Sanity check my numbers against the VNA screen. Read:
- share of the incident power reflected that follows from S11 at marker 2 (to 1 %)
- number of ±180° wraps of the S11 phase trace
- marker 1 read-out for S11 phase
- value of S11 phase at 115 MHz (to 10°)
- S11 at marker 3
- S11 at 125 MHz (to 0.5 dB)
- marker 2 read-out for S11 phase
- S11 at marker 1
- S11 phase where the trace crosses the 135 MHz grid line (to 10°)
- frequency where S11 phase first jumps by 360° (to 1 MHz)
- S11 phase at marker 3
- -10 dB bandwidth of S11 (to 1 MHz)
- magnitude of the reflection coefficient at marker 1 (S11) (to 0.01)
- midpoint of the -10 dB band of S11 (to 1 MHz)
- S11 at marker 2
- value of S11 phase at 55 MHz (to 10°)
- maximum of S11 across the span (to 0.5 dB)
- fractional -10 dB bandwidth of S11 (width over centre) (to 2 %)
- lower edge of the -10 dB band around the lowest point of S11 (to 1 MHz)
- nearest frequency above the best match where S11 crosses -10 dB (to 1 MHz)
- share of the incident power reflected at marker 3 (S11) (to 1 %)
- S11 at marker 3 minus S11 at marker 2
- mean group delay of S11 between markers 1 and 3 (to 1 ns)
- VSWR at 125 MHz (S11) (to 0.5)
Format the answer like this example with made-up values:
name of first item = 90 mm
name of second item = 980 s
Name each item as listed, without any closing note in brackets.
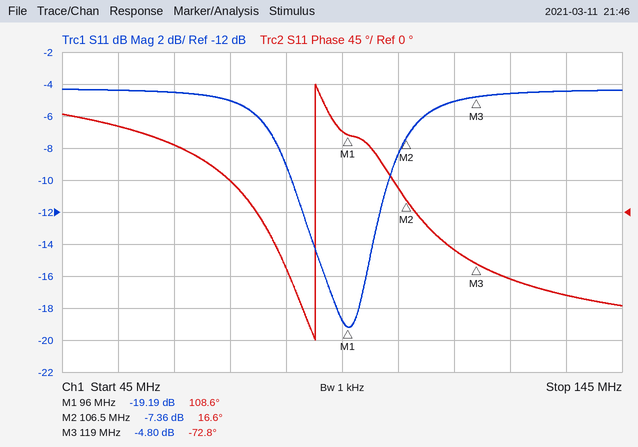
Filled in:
share of the incident power reflected that follows from S11 at marker 2 = 18 %
number of ±180° wraps of the S11 phase trace = 1
marker 1 read-out for S11 phase = 108.6°
value of S11 phase at 115 MHz = -50°
S11 at marker 3 = -4.80 dB
S11 at 125 MHz = -4.5 dB
marker 2 read-out for S11 phase = 16.6°
S11 at marker 1 = -19.19 dB
S11 phase where the trace crosses the 135 MHz grid line = -120°
frequency where S11 phase first jumps by 360° = 90 MHz
S11 phase at marker 3 = -72.8°
-10 dB bandwidth of S11 = 17 MHz
magnitude of the reflection coefficient at marker 1 (S11) = 0.11
midpoint of the -10 dB band of S11 = 95 MHz
S11 at marker 2 = -7.36 dB
value of S11 phase at 55 MHz = 120°
maximum of S11 across the span = -4.5 dB
fractional -10 dB bandwidth of S11 (width over centre) = 18 %
lower edge of the -10 dB band around the lowest point of S11 = 86 MHz
nearest frequency above the best match where S11 crosses -10 dB = 103 MHz
share of the incident power reflected at marker 3 (S11) = 33 %
S11 at marker 3 minus S11 at marker 2 = 2.56 dB
mean group delay of S11 between markers 1 and 3 = 22 ns
VSWR at 125 MHz (S11) = 4.0
